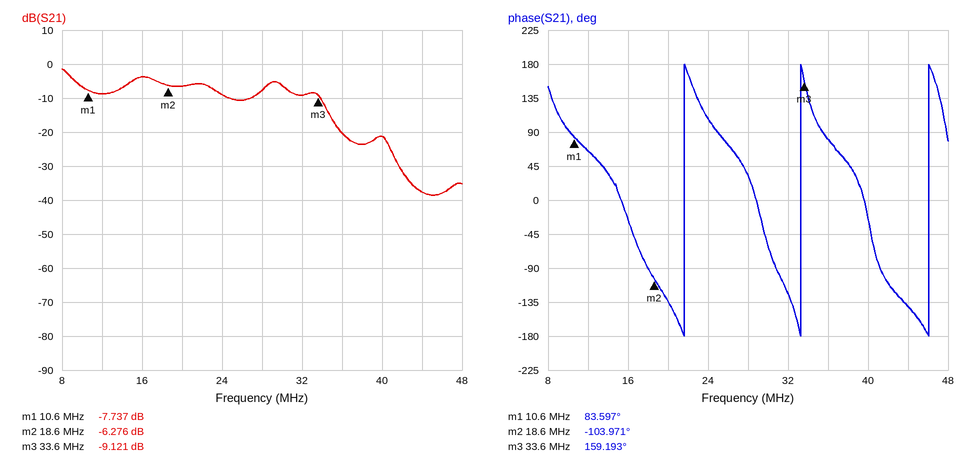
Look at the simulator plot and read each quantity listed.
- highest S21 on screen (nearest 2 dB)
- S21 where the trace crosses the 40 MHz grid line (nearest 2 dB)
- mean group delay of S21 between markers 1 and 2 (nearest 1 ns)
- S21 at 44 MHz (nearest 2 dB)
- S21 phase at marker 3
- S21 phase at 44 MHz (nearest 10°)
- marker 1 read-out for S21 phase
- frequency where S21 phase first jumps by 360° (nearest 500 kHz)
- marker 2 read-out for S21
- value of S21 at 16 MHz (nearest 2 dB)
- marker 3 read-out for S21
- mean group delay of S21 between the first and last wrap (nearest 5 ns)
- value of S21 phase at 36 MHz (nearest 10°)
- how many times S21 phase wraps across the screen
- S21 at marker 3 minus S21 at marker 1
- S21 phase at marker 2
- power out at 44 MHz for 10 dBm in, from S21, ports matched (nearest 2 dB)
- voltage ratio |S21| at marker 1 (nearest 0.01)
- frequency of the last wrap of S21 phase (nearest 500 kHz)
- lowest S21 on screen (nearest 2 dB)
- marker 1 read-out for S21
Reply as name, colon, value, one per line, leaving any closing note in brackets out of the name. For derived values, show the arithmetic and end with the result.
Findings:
highest S21 on screen: -2 dB
S21 where the trace crosses the 40 MHz grid line: -22 dB
mean group delay of S21 between markers 1 and 2: −(-103.971° − (83.597°))/(360° × 8 MHz) ≈ 65 ns
S21 at 44 MHz: -38 dB
S21 phase at marker 3: 159.193°
S21 phase at 44 MHz: -140°
marker 1 read-out for S21 phase: 83.597°
frequency where S21 phase first jumps by 360°: 21.5 MHz
marker 2 read-out for S21: -6.276 dB
value of S21 at 16 MHz: -4 dB
marker 3 read-out for S21: -9.121 dB
mean group delay of S21 between the first and last wrap: 2 cycles / (46.0 MHz − 21.5 MHz) ≈ 81.6 ns, so 80 ns to the nearest 5 ns
value of S21 phase at 36 MHz: 80°
how many times S21 phase wraps across the screen: 3
S21 at marker 3 minus S21 at marker 1: -9.121 − (-7.737) = -1.384 dB
S21 phase at marker 2: -103.971°
power out at 44 MHz for 10 dBm in, from S21, ports matched: 10 dBm + (-38 dB) = -28 dBm
voltage ratio |S21| at marker 1: 10^(-7.737/20) ≈ 0.41
frequency of the last wrap of S21 phase: 46.0 MHz
lowest S21 on screen: -38 dB
marker 1 read-out for S21: -7.737 dB
